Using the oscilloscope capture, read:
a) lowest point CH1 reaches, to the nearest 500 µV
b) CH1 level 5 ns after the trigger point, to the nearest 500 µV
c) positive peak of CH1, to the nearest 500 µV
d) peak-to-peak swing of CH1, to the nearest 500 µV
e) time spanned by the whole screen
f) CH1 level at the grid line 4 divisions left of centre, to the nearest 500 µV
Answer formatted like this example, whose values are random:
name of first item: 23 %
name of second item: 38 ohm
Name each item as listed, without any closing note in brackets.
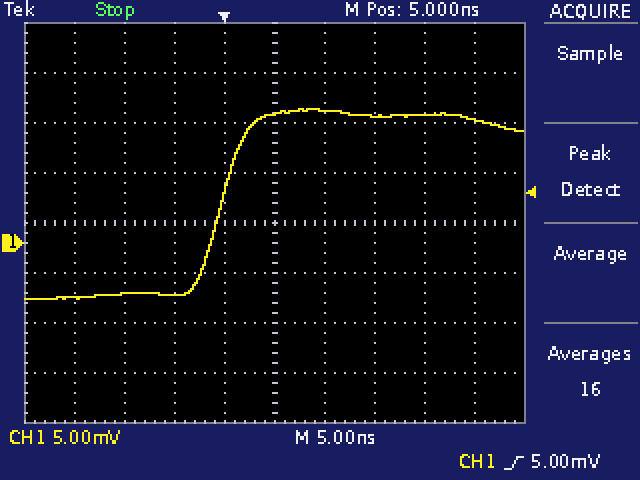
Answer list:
lowest point CH1 reaches, to the nearest 500 µV: -5.5 mV
CH1 level 5 ns after the trigger point, to the nearest 500 µV: 13.0 mV
positive peak of CH1, to the nearest 500 µV: 13.5 mV
peak-to-peak swing of CH1, to the nearest 500 µV: 19.0 mV
time spanned by the whole screen: 50 ns
CH1 level at the grid line 4 divisions left of centre, to the nearest 500 µV: -5.5 mV
